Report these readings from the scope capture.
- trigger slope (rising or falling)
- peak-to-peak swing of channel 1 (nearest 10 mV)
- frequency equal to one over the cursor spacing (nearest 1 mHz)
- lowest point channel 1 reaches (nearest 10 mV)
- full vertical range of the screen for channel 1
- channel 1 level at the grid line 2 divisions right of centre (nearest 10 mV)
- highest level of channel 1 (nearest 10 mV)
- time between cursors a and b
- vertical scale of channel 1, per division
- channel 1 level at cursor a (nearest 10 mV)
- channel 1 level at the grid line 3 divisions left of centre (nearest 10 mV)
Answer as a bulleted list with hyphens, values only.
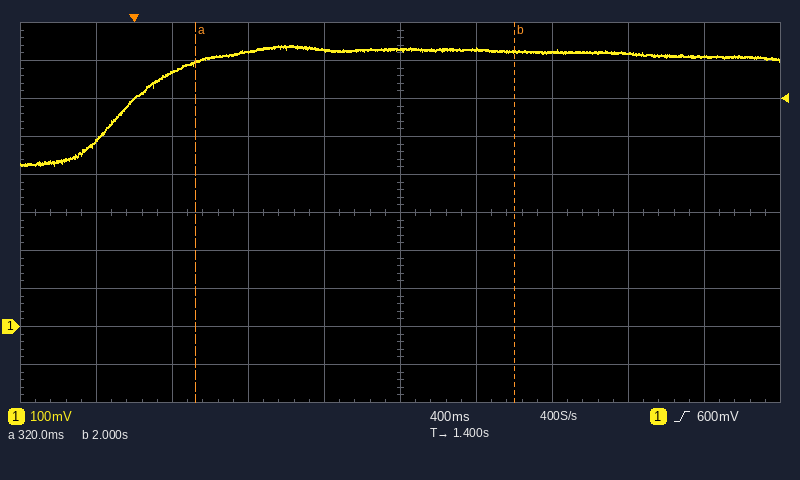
- rising
- 320 mV
- 595 mHz
- 420 mV
- 1 V
- 720 mV
- 740 mV
- 1.68 s
- 100 mV
- 690 mV
- 670 mV
